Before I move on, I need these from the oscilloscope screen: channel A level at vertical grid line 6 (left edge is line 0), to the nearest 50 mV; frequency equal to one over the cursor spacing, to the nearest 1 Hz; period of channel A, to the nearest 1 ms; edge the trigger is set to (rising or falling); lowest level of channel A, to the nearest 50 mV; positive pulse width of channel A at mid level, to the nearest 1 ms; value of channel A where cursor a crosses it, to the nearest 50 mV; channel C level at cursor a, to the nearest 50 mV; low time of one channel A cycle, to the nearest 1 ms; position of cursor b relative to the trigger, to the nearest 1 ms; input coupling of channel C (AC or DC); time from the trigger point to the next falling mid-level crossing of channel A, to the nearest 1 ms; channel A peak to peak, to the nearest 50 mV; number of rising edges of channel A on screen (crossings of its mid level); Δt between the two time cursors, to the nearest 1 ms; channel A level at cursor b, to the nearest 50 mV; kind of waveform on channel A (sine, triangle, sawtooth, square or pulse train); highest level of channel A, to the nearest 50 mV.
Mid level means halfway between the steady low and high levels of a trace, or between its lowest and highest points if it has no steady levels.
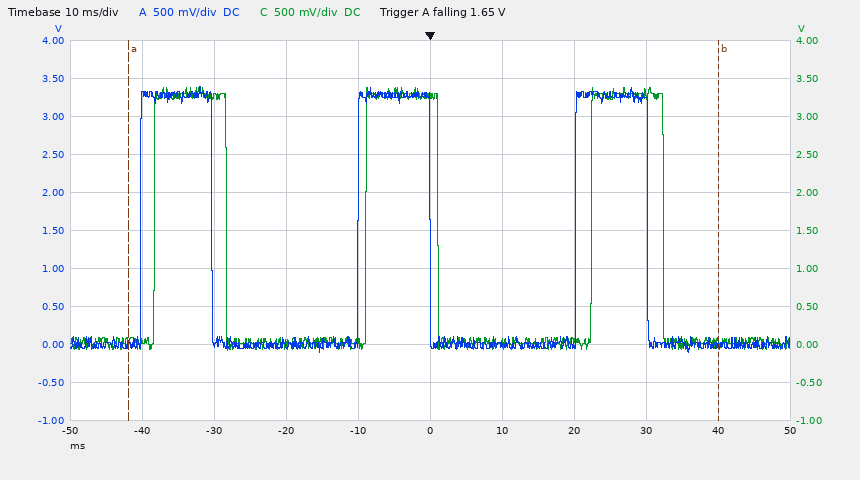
0 mV
12 Hz
30 ms
falling
-100 mV
10 ms
0 mV
50 mV
20 ms
+40 ms
DC
30 ms
3.50 V
3
82 ms
0 mV
pulse train
3.40 V
